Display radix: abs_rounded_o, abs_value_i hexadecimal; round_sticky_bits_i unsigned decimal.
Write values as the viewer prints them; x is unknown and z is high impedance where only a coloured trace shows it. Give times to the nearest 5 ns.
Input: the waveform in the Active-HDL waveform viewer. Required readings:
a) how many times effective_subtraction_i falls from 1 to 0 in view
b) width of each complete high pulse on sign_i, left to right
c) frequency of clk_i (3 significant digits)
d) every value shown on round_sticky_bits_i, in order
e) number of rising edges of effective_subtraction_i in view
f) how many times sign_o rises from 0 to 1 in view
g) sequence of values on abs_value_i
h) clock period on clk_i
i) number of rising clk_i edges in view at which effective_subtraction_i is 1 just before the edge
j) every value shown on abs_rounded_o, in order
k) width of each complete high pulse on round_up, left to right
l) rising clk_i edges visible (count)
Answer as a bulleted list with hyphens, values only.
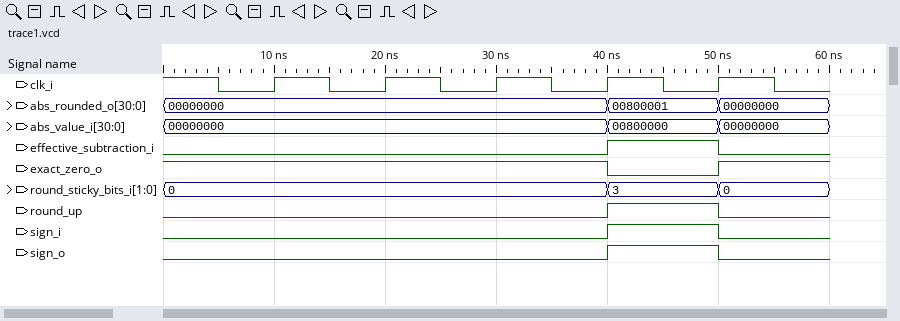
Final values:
- 1
- 10 ns
- 100 MHz
- 0, 3, 0
- 1
- 1
- 00000000, 00800000, 00000000
- 10 ns
- 1
- 00000000, 00800001, 00000000
- 10 ns
- 5
